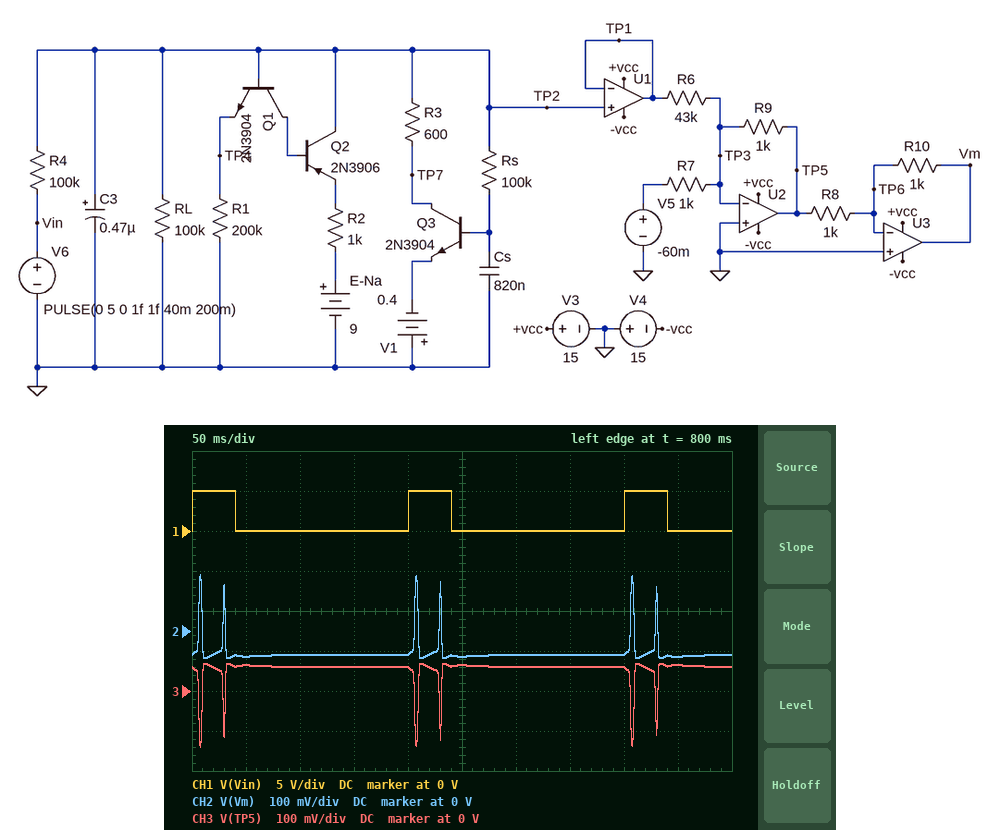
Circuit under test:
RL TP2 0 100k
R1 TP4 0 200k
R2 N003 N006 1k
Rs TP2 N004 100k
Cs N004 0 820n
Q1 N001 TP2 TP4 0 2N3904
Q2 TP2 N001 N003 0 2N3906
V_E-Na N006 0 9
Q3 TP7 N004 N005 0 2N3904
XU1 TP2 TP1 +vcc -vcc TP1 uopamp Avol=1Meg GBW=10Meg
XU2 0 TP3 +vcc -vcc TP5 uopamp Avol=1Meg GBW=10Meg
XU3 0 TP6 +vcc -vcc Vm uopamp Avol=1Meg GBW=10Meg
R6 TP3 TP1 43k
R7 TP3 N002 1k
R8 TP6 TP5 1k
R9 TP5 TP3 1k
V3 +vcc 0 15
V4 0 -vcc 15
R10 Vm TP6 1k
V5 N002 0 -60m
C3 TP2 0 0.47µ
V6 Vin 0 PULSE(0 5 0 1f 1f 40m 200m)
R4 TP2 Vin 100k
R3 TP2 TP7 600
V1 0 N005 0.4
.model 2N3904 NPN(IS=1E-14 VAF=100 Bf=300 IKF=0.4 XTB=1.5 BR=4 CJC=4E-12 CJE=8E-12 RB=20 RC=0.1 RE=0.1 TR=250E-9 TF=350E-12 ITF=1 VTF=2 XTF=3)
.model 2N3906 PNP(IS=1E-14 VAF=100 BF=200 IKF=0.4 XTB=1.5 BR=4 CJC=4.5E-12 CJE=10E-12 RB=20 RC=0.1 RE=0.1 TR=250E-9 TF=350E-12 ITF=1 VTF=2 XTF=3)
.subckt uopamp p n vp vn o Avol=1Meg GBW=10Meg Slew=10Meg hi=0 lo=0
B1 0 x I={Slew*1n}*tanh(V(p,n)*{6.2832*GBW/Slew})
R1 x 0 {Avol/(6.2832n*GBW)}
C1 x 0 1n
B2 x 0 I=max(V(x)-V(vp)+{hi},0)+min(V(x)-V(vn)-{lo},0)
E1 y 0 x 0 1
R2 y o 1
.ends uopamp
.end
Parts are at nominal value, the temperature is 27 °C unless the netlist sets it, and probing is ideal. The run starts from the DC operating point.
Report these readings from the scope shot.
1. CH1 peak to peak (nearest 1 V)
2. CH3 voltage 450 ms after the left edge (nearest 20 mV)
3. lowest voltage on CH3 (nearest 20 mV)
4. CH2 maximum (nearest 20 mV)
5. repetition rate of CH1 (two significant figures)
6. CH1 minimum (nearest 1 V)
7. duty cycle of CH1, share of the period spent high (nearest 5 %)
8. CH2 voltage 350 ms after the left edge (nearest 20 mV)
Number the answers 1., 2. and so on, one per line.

1. 5 V
2. 60 mV
3. -140 mV
4. 140 mV
5. 5.0 Hz
6. 0 V
7. 20 %
8. -60 mV
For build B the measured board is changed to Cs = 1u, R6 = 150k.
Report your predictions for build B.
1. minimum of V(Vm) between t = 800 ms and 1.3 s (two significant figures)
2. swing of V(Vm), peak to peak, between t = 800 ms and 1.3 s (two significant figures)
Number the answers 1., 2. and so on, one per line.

1. -62 mV
2. 60 mV
